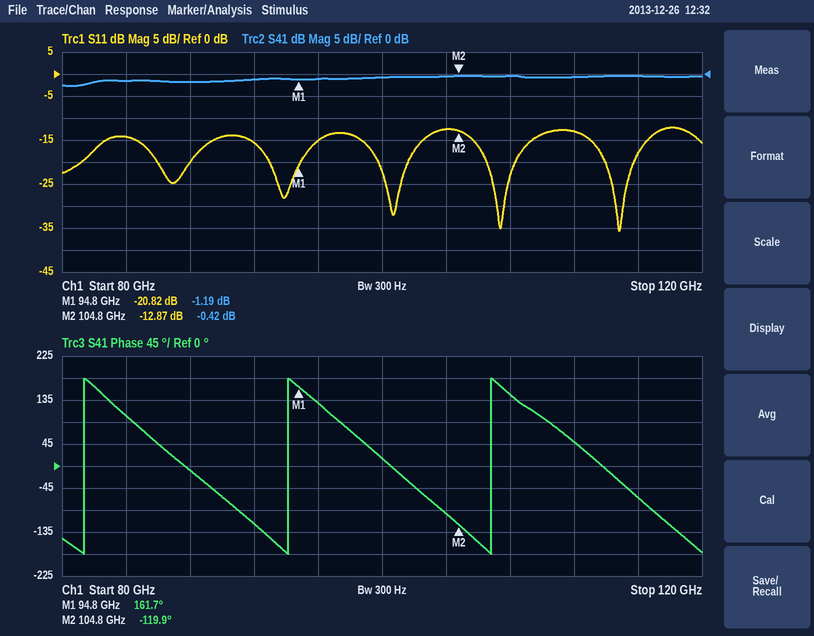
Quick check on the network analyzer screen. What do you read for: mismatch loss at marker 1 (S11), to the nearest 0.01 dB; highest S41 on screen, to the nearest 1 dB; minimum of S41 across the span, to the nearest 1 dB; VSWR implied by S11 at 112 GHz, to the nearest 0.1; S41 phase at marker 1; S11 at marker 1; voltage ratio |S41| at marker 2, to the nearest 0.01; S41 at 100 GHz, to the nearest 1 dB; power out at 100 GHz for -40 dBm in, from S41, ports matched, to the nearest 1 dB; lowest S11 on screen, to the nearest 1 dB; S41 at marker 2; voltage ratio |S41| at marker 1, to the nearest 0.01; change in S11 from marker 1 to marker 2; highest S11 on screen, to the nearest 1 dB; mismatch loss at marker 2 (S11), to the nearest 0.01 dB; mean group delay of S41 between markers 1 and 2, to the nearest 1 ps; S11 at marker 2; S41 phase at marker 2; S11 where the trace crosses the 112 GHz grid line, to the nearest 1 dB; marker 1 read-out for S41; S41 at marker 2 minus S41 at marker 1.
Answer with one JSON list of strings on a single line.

["0.04 dB", "0 dB", "-3 dB", "1.6", "161.7°", "-20.82 dB", "0.95", "-1 dB", "-41 dBm", "-36 dB", "-0.42 dB", "0.87", "7.95 dB", "-12 dB", "0.23 dB", "78 ps", "-12.87 dB", "-119.9°", "-13 dB", "-1.19 dB", "0.77 dB"]
